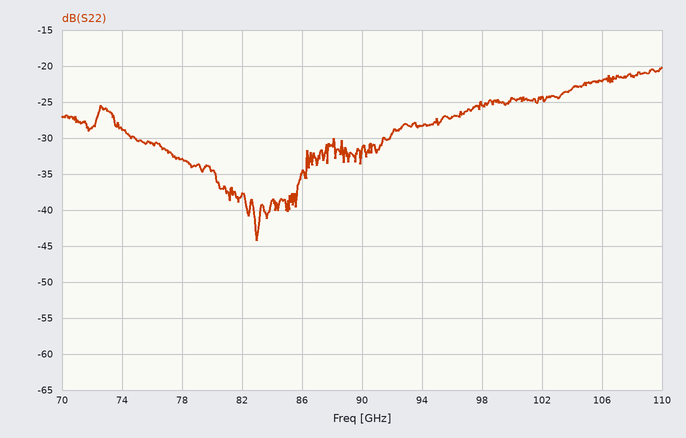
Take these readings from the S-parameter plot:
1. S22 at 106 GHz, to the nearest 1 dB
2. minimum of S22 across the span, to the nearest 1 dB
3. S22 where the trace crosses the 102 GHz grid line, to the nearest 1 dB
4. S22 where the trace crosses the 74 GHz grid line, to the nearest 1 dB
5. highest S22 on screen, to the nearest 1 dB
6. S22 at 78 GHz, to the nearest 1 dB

-22 dB
-44 dB
-24 dB
-29 dB
-20 dB
-33 dB
